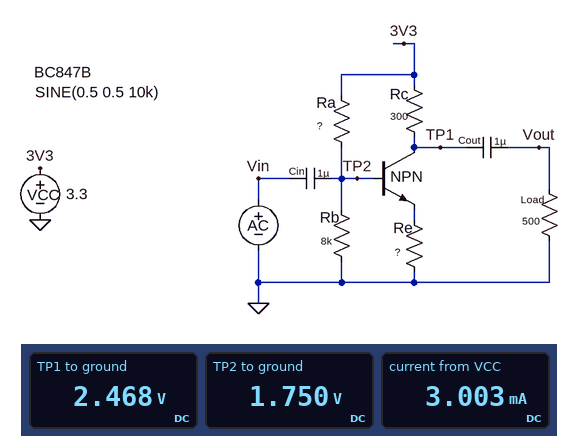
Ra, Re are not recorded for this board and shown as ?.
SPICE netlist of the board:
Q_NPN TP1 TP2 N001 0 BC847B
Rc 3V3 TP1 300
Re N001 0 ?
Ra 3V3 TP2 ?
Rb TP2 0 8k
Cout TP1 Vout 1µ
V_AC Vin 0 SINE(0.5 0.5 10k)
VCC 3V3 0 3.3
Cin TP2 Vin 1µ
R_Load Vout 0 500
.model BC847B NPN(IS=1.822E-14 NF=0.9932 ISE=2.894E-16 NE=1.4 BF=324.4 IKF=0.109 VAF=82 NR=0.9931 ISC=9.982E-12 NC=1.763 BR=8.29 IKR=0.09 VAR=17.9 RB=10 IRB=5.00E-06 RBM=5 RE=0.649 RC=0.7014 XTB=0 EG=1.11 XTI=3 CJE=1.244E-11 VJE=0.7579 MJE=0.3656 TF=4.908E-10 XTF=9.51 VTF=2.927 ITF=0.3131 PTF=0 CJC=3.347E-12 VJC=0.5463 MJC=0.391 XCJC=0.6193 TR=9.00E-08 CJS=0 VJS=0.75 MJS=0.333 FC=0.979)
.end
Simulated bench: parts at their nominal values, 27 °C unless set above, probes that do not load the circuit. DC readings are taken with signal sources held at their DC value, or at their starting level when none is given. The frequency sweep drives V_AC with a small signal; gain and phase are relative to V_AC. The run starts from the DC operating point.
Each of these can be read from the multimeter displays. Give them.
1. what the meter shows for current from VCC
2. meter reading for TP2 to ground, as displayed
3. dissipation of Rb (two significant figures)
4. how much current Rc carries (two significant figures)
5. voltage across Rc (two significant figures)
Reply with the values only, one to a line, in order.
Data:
3.003 mA
1.750 V
380 µW
2.8 mA
830 mV
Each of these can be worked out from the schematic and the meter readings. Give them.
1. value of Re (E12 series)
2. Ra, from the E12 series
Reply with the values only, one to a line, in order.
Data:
390 Ω
6.8 kΩ
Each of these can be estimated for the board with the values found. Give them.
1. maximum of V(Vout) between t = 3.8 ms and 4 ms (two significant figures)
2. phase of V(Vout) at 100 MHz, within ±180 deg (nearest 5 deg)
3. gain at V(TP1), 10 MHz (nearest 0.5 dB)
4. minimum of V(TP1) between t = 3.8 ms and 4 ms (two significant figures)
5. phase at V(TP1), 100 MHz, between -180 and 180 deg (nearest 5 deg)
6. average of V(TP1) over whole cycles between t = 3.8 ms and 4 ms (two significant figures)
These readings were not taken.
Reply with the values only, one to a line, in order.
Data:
230 mV
115 deg
-6.5 dB
2.2 V
115 deg
2.5 V
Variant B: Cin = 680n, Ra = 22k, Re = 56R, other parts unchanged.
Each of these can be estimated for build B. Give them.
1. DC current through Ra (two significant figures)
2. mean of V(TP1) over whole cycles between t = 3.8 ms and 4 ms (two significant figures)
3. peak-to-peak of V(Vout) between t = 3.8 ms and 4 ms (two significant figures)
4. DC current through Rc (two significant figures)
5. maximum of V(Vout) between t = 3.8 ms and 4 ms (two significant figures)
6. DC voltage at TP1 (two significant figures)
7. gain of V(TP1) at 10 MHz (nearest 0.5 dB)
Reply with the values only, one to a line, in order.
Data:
110 µA
2.1 V
2.0 V
2.9 mA
770 mV
2.4 V
9.0 dB
